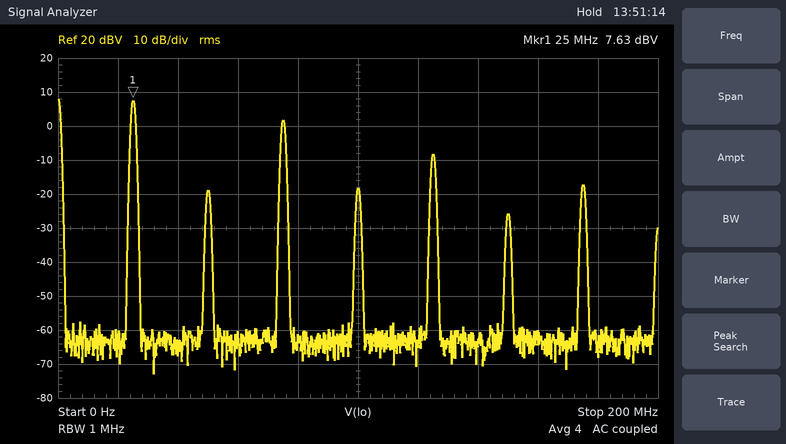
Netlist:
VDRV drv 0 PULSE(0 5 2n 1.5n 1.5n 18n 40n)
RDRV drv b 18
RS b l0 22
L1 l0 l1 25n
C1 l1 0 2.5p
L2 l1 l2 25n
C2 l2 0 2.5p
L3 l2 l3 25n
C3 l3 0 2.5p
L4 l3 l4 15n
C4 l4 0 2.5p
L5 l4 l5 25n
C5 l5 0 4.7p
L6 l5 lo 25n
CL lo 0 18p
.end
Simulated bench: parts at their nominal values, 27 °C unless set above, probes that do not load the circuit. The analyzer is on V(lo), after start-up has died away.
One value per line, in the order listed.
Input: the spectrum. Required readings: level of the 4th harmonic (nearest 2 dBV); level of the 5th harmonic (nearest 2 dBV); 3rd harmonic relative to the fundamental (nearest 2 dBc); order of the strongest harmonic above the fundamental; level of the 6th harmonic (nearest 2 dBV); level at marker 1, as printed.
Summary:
-18 dBV
-8 dBV
-6 dBc
3
-26 dBV
7.63 dBV
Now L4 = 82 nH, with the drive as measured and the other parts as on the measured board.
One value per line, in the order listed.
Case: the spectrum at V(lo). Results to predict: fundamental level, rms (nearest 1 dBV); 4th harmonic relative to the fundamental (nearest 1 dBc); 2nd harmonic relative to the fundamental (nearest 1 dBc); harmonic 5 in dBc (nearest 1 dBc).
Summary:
8 dBV
-29 dBc
-25 dBc
-20 dBc
